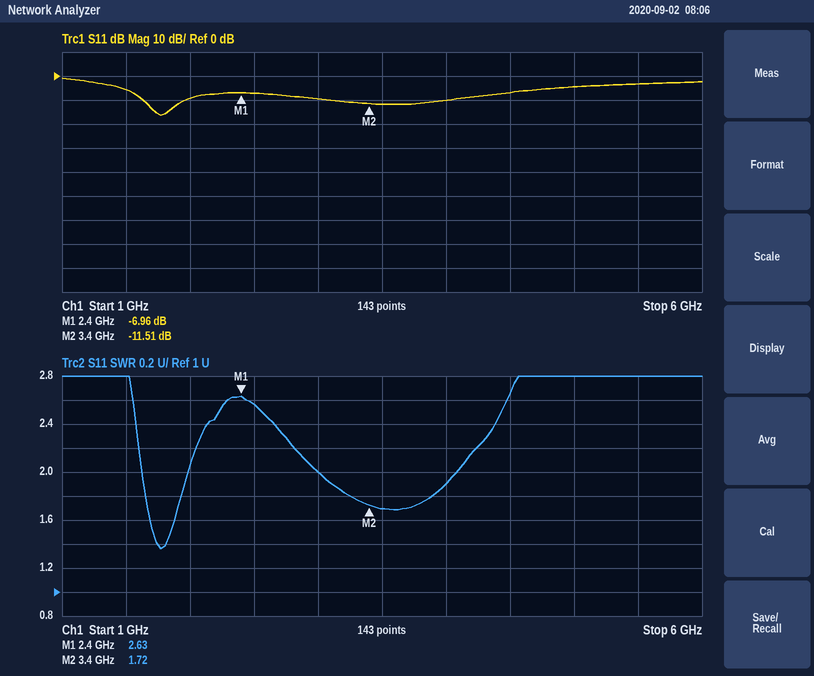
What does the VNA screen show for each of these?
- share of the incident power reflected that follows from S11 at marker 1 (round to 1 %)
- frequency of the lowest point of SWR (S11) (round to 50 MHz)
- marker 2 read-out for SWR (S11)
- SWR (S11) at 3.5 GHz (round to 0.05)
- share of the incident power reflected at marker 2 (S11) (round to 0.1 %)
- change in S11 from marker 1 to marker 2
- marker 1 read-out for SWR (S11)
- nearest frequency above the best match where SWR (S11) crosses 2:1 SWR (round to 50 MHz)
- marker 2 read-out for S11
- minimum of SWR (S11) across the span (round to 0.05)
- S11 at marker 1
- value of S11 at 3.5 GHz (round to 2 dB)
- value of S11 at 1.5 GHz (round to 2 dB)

20 %
1.75 GHz
1.72
1.70
7.1 %
-4.55 dB
2.63
2.00 GHz
-11.51 dB
1.35
-6.96 dB
-12 dB
-6 dB
